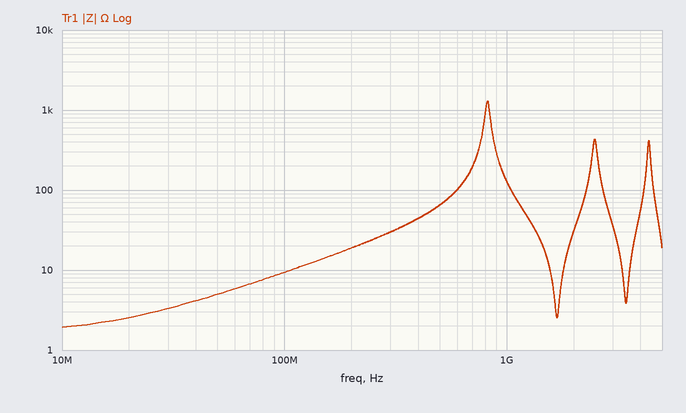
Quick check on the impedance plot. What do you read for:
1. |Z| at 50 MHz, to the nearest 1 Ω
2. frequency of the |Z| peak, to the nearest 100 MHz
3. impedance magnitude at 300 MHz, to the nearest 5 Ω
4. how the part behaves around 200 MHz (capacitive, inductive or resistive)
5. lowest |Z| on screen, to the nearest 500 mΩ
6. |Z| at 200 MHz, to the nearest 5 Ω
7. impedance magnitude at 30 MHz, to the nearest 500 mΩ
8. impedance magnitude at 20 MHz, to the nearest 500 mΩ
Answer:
5 Ω
800 MHz
30 Ω
inductive
2.0 Ω
20 Ω
3.5 Ω
2.5 Ω
